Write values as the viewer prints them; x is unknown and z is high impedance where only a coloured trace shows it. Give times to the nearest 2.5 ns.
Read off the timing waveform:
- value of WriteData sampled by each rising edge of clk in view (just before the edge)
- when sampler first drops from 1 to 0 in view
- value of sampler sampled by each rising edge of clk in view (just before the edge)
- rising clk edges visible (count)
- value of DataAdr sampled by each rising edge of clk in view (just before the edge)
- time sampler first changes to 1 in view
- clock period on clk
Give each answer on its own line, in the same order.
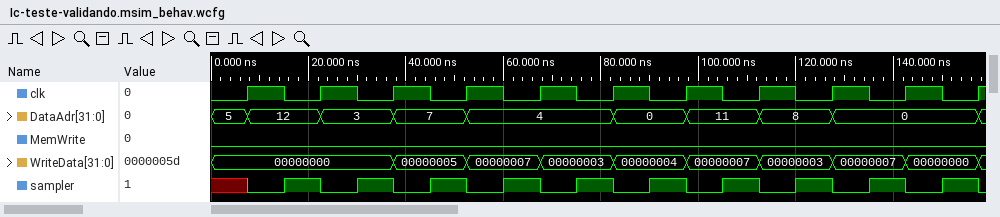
00000000, 00000000, 00000000, 00000005, 00000007, 00000003, 00000004, 00000007, 00000003, 00000007, 00000000
22.5 ns
x 1 1 1 1 1 1 1 1 1 1
11
5, 12, 3, 7, 4, 4, 0, 11, 8, 0, 0
15 ns
15 ns
